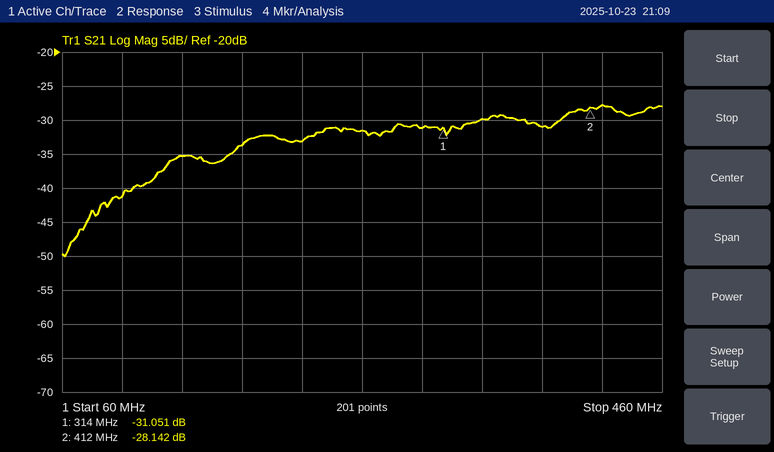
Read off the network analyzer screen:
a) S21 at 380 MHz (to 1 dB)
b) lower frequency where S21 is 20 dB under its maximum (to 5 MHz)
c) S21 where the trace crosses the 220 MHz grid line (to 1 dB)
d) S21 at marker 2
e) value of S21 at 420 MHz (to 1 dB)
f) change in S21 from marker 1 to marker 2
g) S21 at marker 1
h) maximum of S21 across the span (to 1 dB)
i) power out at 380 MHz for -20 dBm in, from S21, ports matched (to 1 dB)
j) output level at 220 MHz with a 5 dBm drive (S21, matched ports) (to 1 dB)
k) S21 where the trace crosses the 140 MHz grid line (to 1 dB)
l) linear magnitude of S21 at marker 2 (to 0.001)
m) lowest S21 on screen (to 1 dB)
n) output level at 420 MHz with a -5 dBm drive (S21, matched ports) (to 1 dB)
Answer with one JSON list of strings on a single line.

["-31 dB", "65 MHz", "-33 dB", "-28.142 dB", "-28 dB", "2.909 dB", "-31.051 dB", "-28 dB", "-51 dBm", "-28 dBm", "-35 dB", "0.039", "-50 dB", "-33 dBm"]
